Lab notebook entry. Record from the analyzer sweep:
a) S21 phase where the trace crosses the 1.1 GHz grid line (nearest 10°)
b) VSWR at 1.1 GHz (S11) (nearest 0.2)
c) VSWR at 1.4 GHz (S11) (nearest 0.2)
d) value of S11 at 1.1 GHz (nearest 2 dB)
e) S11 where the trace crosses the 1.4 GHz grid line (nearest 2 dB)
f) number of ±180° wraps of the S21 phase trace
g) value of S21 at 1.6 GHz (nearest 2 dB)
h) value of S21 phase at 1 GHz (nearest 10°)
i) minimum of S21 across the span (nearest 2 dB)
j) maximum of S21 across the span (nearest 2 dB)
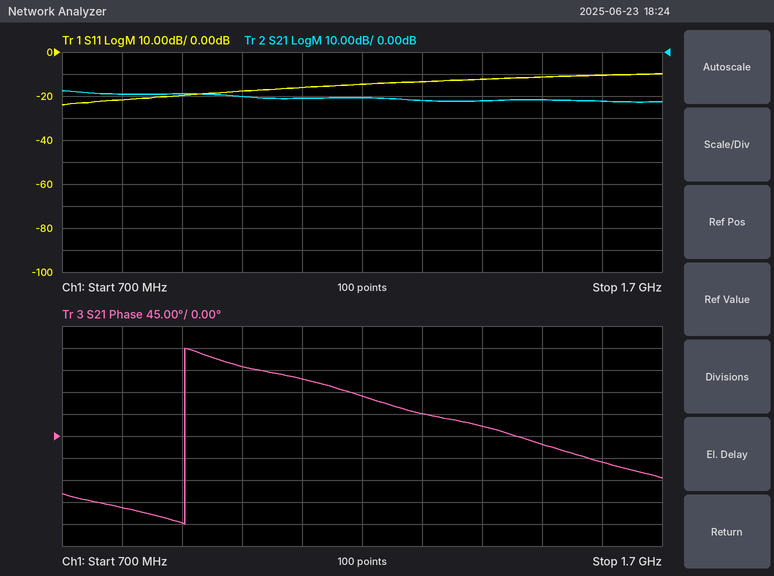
120°
1.4
1.6
-16 dB
-12 dB
1
-22 dB
140°
-22 dB
-18 dB
